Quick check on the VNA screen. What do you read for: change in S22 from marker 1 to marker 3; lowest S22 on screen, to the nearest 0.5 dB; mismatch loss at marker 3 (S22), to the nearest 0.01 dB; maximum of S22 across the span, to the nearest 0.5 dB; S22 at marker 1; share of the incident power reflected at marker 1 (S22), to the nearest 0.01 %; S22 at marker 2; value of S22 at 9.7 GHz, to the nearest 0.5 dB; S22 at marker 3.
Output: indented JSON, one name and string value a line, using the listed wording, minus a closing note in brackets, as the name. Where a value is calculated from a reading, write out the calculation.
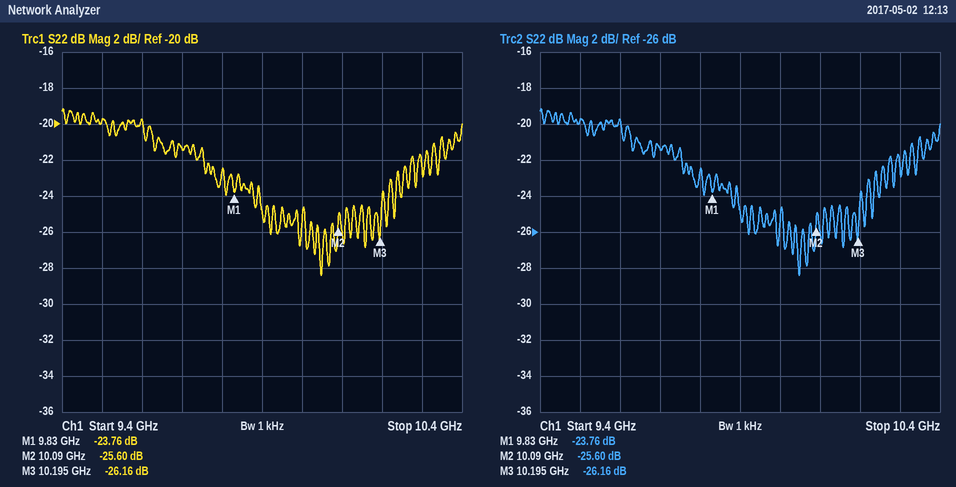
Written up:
{
  "change in S22 from marker 1 to marker 3": "-26.16 − (-23.76) = -2.40 dB",
  "lowest S22 on screen, to the nearest 0.5 dB": "-28.5 dB",
  "mismatch loss at marker 3 (S22), to the nearest 0.01 dB": "−10 log10(1 − 10^(-26.16/10)) ≈ 0.01 dB",
  "maximum of S22 across the span, to the nearest 0.5 dB": "-19.0 dB",
  "S22 at marker 1": "-23.76 dB",
  "share of the incident power reflected at marker 1 (S22), to the nearest 0.01 %": "10^(-23.76/10) ≈ 0.42 %",
  "S22 at marker 2": "-25.60 dB",
  "value of S22 at 9.7 GHz, to the nearest 0.5 dB": "-21.5 dB",
  "S22 at marker 3": "-26.16 dB"
}
